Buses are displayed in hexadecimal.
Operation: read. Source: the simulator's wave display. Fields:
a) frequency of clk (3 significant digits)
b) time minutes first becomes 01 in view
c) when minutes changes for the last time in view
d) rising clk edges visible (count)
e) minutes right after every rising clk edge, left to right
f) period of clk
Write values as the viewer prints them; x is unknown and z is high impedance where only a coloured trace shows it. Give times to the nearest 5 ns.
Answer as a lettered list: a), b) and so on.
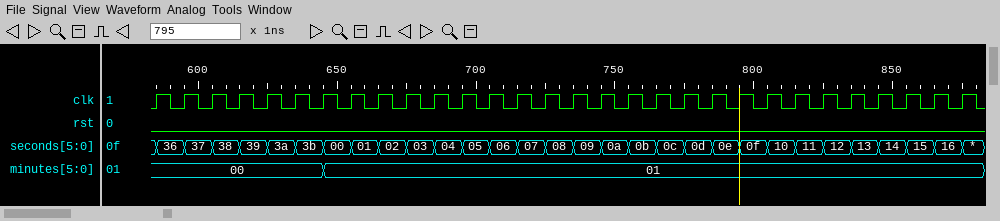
a) 100 MHz
b) 645 ns
c) 645 ns
d) 30
e) 00, 00, 00, 00, 00, 00, 01, 01, 01, 01, 01, 01, 01, 01, 01, 01, 01, 01, 01, 01, 01, 01, 01, 01, 01, 01, 01, 01, 01, 01
f) 10 ns
